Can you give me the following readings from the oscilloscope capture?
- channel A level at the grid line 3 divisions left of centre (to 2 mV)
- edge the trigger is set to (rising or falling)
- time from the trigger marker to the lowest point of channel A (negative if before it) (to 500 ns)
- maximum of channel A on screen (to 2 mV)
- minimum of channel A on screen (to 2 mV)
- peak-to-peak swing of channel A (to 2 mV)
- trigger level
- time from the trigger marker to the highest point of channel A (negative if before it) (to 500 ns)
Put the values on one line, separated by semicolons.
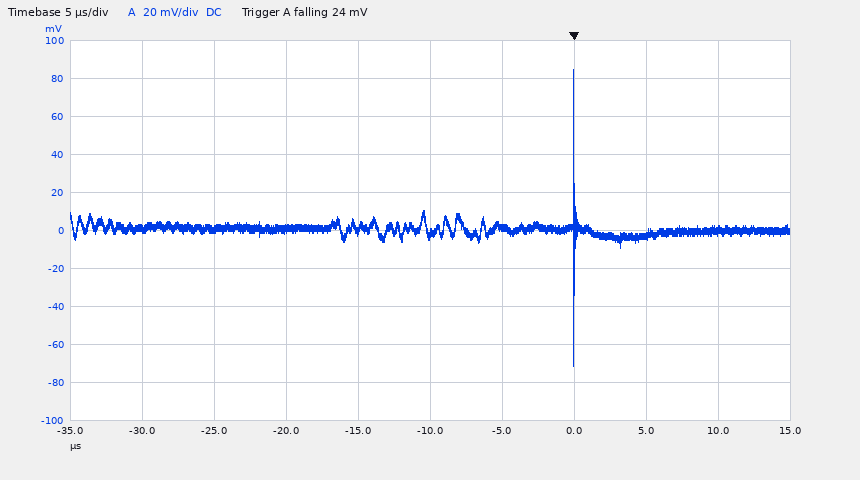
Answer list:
2 mV; falling; 0.0 µs; 84 mV; -72 mV; 156 mV; 24 mV; 0.0 µs
